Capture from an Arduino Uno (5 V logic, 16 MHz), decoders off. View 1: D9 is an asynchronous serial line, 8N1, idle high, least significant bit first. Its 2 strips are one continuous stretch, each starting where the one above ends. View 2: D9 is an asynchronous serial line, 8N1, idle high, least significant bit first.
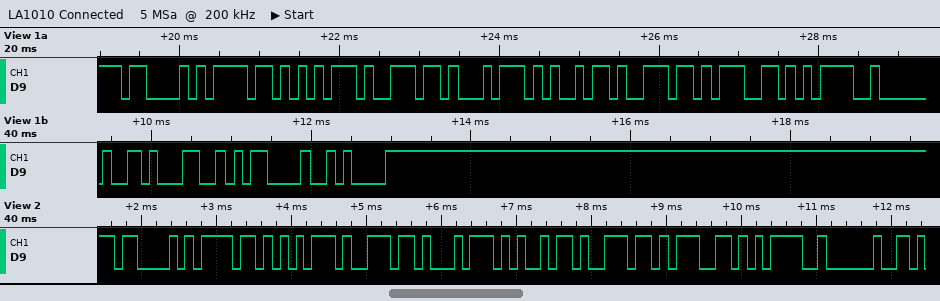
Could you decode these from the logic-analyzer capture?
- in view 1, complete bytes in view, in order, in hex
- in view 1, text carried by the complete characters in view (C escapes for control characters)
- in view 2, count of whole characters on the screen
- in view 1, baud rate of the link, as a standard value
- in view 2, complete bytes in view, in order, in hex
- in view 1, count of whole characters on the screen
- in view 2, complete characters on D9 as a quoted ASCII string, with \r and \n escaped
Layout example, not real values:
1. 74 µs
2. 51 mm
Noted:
1. 0x43 0x6F 0x75 0x6E 0x74 0x69 0x6E 0x67 0x3D 0x20 0x31 0x0D 0x0A
2. "Counting= 1\r\n"
3. 10
4. 9600 baud
5. 0x43 0x6F 0x75 0x6E 0x74 0x69 0x6E 0x67 0x3D 0x20
6. 13
7. "Counting= "
